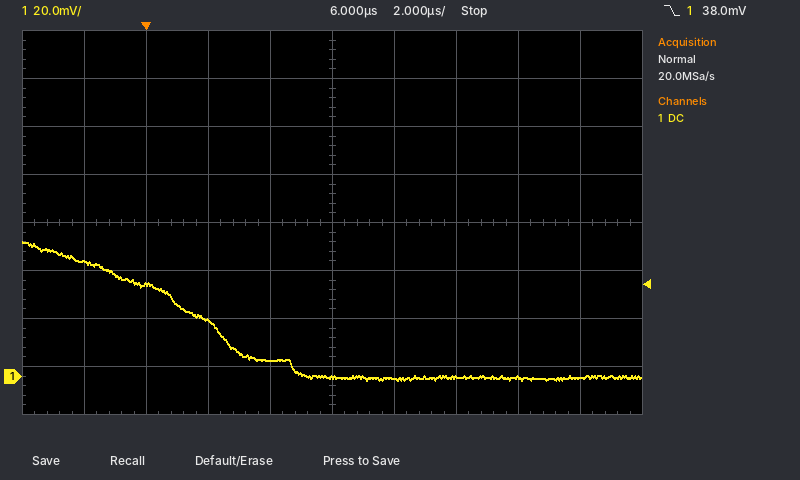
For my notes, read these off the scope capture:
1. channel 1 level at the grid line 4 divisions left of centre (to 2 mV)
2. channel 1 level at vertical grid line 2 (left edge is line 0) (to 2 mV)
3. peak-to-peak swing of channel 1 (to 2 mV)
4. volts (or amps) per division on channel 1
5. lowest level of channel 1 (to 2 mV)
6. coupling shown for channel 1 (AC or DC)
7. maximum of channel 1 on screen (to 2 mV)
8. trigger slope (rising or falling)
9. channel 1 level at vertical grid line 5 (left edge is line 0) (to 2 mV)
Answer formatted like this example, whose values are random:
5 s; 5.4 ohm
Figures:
48 mV; 38 mV; 58 mV; 20 mV; -2 mV; DC; 56 mV; falling; 0 mV
